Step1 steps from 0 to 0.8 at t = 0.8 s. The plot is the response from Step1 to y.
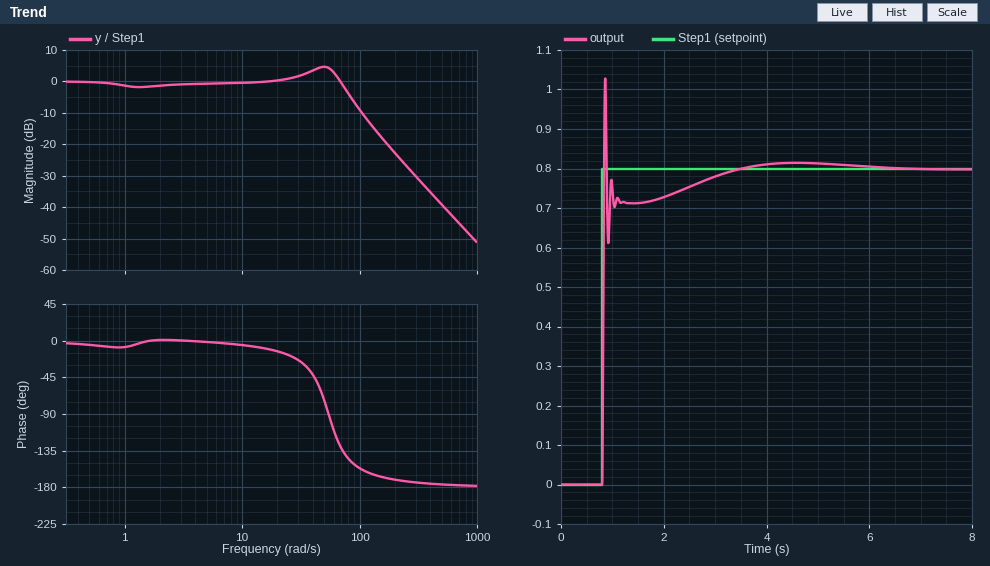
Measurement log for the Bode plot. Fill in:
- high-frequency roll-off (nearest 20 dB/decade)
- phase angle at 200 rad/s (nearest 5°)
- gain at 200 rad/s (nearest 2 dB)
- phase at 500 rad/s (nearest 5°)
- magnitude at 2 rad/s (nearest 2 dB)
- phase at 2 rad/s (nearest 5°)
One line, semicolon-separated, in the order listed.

-40 dB/decade; -170°; -22 dB; -175°; -2 dB; 0°
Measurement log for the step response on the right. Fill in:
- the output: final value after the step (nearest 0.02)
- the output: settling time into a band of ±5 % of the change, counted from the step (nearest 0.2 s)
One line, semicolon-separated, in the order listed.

0.80; 1.8 s
